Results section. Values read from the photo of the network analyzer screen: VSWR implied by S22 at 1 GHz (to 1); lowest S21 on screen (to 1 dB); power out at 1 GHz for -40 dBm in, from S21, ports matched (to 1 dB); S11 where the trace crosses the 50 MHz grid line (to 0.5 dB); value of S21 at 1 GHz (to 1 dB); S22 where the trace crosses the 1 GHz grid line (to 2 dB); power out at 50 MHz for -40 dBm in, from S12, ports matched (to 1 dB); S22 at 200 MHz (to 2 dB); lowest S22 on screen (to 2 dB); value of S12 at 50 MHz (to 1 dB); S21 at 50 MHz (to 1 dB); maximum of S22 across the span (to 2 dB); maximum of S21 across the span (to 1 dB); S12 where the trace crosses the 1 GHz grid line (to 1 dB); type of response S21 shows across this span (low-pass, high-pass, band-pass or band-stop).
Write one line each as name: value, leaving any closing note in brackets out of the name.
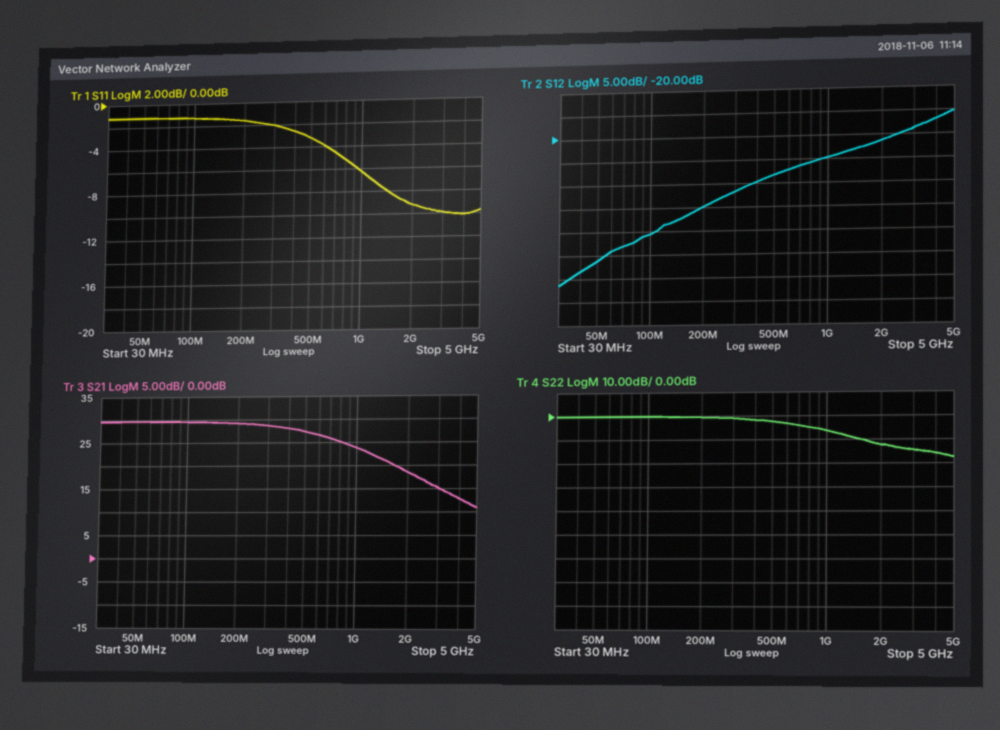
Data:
VSWR implied by S22 at 1 GHz: 3
lowest S21 on screen: 11 dB
power out at 1 GHz for -40 dBm in, from S21, ports matched: -16 dBm
S11 where the trace crosses the 50 MHz grid line: -1.0 dB
value of S21 at 1 GHz: 24 dB
S22 where the trace crosses the 1 GHz grid line: -6 dB
power out at 50 MHz for -40 dBm in, from S12, ports matched: -86 dBm
S22 at 200 MHz: 0 dB
lowest S22 on screen: -18 dB
value of S12 at 50 MHz: -46 dB
S21 at 50 MHz: 30 dB
maximum of S22 across the span: 0 dB
maximum of S21 across the span: 30 dB
S12 where the trace crosses the 1 GHz grid line: -25 dB
type of response S21 shows across this span: low-pass
